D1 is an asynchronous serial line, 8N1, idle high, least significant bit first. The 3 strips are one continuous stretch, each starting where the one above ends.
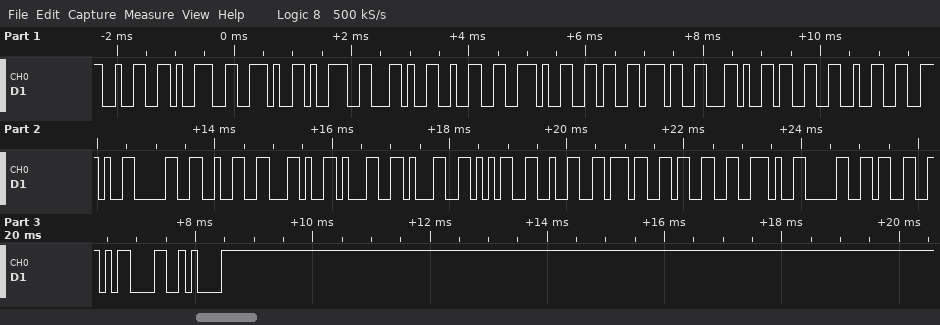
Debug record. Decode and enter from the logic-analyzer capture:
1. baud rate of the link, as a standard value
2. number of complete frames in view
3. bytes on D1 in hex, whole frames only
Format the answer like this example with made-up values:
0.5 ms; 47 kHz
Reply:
9600 baud; 27; 32 39 2E 39 2C 32 2E 36 37 2C 33 32 2E 30 32 2C 31 31 35 32 37 33 2E 30 33 0D 0A
